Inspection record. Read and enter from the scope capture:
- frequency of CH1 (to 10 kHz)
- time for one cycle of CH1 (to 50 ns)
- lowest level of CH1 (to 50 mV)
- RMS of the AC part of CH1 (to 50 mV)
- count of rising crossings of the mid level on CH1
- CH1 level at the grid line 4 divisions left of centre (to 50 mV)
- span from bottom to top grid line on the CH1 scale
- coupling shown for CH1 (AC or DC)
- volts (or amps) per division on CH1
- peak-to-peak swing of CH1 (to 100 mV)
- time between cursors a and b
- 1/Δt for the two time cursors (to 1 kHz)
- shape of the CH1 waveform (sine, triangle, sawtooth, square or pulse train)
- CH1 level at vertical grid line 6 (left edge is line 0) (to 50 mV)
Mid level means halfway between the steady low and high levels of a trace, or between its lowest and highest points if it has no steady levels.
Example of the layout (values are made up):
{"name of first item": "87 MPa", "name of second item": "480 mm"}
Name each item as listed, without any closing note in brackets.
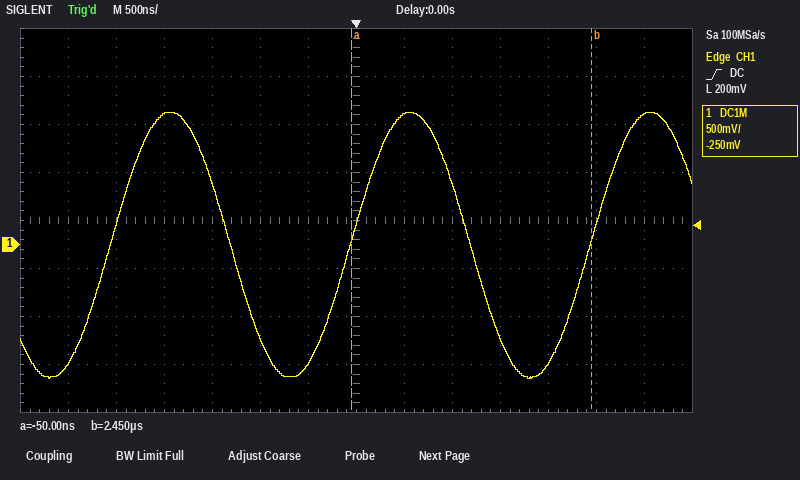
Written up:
{"frequency of CH1": "400 kHz", "time for one cycle of CH1": "2.50 µs", "lowest level of CH1": "-1.40 V", "RMS of the AC part of CH1": "1.00 V", "count of rising crossings of the mid level on CH1": "3", "CH1 level at the grid line 4 divisions left of centre": "1.35 V", "span from bottom to top grid line on the CH1 scale": "4 V", "coupling shown for CH1": "DC", "volts (or amps) per division on CH1": "500 mV", "peak-to-peak swing of CH1": "2.80 V", "time between cursors a and b": "2.50 µs", "1/Δt for the two time cursors": "400 kHz", "shape of the CH1 waveform": "sine", "CH1 level at vertical grid line 6 (left edge is line 0)": "-1.25 V"}
